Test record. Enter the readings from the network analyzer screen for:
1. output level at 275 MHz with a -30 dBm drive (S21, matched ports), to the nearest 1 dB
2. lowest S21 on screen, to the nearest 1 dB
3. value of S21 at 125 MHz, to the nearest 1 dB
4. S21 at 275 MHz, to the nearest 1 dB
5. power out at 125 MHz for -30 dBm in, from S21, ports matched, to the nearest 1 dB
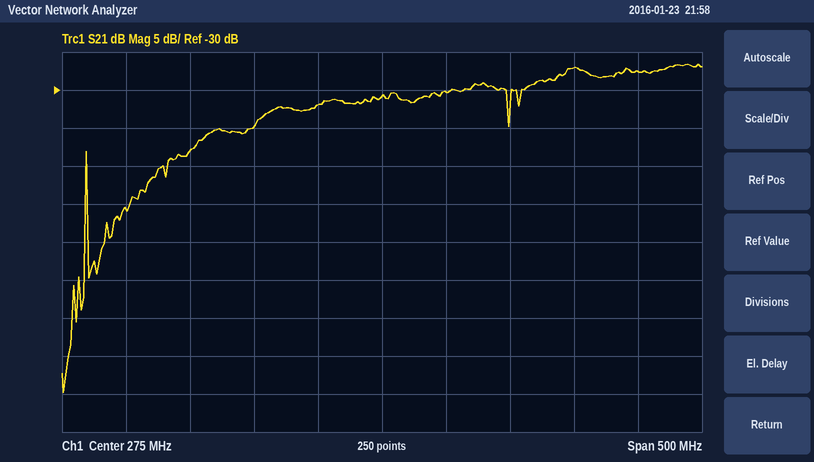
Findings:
-61 dBm
-70 dB
-38 dB
-31 dB
-68 dBm
